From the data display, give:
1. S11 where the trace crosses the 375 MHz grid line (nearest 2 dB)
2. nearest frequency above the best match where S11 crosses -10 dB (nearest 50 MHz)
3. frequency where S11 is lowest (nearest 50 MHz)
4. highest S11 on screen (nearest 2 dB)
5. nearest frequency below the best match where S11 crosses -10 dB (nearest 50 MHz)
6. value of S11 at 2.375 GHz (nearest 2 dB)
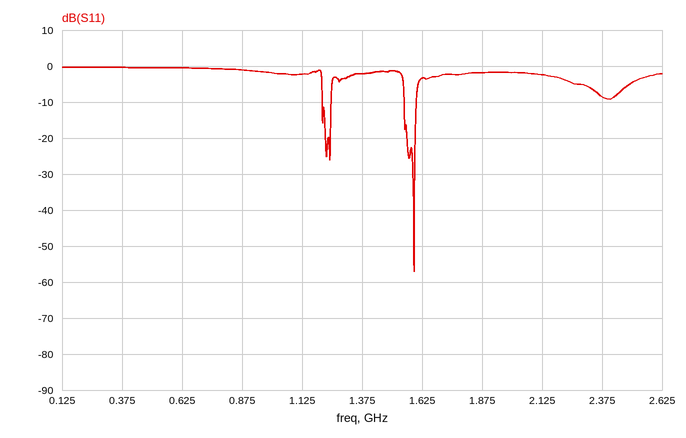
0 dB
1.60 GHz
1.60 GHz
0 dB
1.55 GHz
-8 dB
